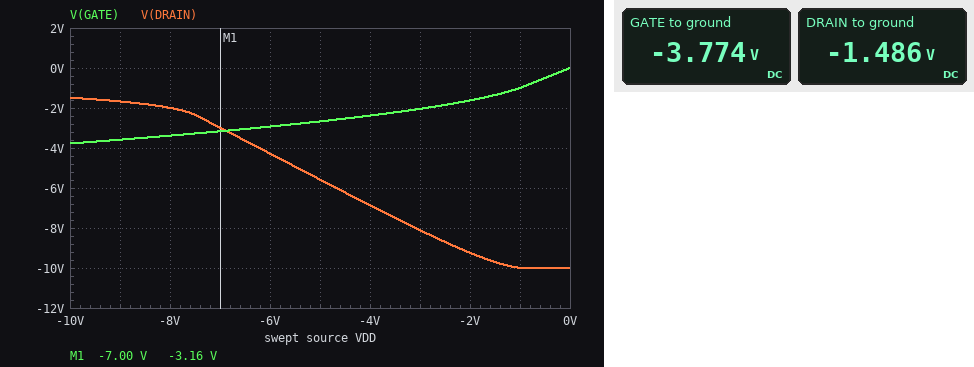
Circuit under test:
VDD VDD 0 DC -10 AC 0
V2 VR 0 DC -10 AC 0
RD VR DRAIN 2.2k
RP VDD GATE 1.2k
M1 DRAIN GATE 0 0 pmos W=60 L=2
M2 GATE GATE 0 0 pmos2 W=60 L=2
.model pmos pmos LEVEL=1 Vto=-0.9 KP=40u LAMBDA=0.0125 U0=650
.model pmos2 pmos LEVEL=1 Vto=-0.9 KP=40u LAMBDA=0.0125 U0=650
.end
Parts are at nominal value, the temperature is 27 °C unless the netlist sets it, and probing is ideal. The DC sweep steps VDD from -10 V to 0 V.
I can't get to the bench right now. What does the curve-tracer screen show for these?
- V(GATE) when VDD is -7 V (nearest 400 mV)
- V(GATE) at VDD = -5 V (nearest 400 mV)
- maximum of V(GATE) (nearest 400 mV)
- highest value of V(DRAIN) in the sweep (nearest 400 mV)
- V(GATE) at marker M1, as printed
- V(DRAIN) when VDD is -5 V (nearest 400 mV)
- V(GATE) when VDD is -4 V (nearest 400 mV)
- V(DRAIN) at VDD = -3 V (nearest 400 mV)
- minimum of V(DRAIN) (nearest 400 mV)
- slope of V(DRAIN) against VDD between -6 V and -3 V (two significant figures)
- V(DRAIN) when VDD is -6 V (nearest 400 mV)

-3.2 V
-2.8 V
0 V
-1.6 V
-3.16 V
-5.6 V
-2.4 V
-8.0 V
-10.0 V
-1.3 V/V
-4.4 V
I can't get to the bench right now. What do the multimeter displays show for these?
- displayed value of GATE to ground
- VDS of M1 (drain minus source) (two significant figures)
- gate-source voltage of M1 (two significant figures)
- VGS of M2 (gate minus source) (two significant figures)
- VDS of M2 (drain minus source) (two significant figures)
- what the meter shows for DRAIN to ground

-3.774 V
-1.5 V
-3.8 V
-3.8 V
-3.8 V
-1.486 V
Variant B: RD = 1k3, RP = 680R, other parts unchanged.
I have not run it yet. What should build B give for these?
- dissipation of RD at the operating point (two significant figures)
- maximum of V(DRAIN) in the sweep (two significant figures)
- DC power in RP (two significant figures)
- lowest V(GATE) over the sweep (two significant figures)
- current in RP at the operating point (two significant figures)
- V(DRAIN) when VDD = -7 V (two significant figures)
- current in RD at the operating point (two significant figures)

50 mW
-1.9 V
45 mW
-4.5 V
8.1 mA
-3.7 V
6.2 mA
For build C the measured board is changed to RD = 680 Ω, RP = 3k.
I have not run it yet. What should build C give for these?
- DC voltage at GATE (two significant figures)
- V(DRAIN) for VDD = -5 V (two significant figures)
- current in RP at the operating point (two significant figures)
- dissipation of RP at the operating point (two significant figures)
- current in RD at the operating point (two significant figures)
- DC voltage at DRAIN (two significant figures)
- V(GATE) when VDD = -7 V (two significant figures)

-2.9 V
-9.3 V
2.4 mA
17 mW
2.5 mA
-8.3 V
-2.5 V
